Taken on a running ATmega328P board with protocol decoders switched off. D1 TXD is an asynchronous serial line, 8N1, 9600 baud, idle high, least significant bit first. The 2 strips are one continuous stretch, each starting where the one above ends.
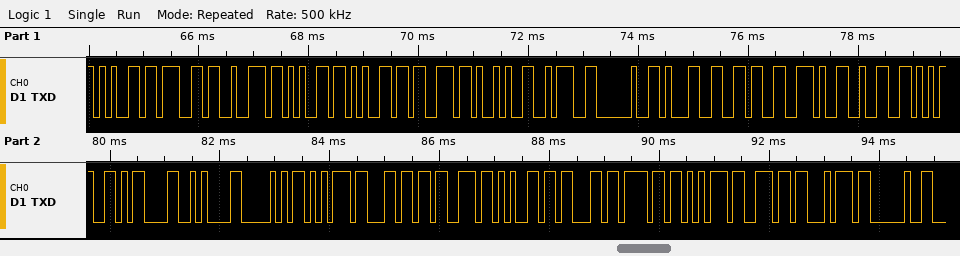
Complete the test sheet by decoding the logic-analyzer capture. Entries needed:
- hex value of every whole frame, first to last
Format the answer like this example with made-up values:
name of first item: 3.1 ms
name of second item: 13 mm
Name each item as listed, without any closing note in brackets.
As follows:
hex value of every whole frame, first to last: 65 67 72 65 65 73 29 3A 20 31 36 2E 32 35 0D 0A 50 75 6C 73 65 63 6F 75 6E 74 20
